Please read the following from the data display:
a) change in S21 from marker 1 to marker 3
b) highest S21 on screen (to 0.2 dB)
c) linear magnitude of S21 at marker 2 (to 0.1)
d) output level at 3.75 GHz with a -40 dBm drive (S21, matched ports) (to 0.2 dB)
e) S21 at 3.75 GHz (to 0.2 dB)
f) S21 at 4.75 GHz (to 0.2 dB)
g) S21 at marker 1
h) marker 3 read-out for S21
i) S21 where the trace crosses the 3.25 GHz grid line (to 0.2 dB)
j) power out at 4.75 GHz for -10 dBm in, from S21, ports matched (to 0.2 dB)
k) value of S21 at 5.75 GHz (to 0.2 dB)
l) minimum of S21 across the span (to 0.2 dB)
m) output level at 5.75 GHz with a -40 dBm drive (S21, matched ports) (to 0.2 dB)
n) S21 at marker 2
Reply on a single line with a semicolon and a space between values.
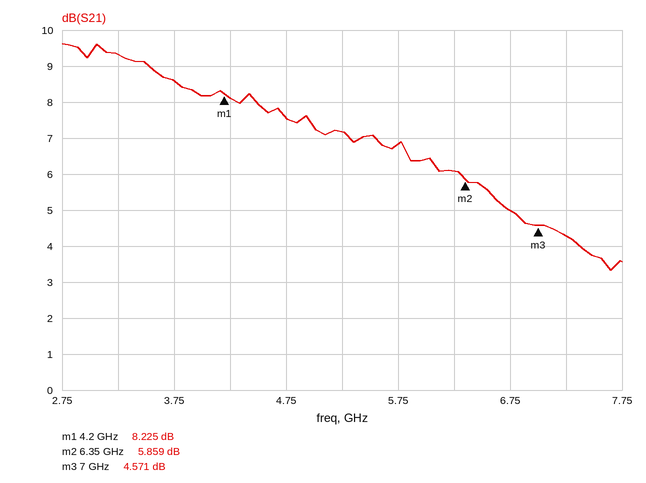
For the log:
-3.654 dB; 9.6 dB; 2.0; -31.4 dBm; 8.6 dB; 7.6 dB; 8.225 dB; 4.571 dB; 9.4 dB; -2.4 dBm; 6.8 dB; 3.4 dB; -33.2 dBm; 5.859 dB
